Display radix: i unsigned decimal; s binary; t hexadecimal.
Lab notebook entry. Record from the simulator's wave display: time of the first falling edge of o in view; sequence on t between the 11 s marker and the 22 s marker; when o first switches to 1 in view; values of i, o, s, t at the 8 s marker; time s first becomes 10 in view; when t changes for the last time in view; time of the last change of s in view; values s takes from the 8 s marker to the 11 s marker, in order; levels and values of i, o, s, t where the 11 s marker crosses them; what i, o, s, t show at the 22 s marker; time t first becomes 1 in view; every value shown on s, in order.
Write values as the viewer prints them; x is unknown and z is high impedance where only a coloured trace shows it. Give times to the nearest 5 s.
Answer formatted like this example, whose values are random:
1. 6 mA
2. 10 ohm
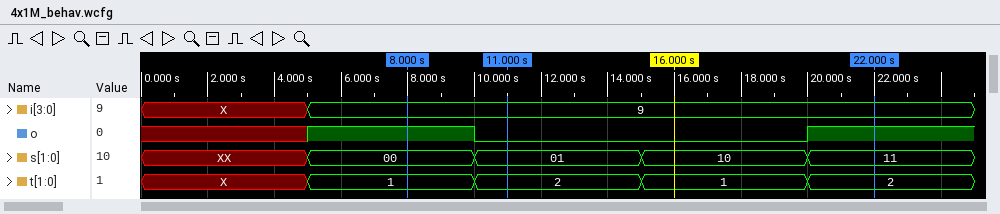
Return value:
1. 10 s
2. 2, 1, 2
3. 5 s
4. i=9, o=1, s=00, t=1
5. 15 s
6. 20 s
7. 20 s
8. 00, 01
9. i=9, o=0, s=01, t=2
10. i=9, o=1, s=11, t=2
11. 5 s
12. XX, 00, 01, 10, 11
